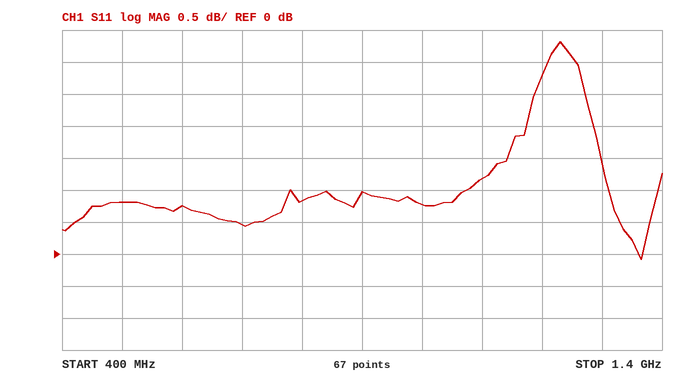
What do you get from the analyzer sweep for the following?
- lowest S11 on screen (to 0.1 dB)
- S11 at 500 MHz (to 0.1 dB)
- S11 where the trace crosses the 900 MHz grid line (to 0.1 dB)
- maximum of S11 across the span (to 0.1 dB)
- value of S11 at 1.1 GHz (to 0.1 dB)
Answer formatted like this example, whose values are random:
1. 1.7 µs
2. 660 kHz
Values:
1. -0.1 dB
2. 0.8 dB
3. 1.0 dB
4. 3.3 dB
5. 1.2 dB
